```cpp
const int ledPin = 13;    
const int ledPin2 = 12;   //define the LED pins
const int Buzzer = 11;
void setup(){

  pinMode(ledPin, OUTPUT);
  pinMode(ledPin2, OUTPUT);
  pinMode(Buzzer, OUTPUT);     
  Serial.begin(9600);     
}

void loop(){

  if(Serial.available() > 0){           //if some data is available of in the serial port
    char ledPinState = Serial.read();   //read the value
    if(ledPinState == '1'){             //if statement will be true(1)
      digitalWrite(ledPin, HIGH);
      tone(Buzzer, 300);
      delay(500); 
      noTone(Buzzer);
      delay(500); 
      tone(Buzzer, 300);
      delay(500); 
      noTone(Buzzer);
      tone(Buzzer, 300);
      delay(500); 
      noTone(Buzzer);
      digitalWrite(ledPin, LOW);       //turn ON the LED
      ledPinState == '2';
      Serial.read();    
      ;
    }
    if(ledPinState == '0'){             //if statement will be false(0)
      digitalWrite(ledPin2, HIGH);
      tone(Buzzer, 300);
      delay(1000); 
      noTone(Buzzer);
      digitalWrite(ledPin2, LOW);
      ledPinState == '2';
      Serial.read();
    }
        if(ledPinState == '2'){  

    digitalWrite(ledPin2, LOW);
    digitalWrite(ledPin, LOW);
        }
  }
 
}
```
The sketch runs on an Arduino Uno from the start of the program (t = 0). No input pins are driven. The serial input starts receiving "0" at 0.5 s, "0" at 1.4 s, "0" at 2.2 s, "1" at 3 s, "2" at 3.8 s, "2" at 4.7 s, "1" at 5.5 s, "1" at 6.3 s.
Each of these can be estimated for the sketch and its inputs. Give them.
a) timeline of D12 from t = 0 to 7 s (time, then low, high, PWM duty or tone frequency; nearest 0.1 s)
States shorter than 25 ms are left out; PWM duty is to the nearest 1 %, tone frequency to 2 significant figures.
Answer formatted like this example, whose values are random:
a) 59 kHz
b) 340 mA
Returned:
a) 0 s low; 0.5 s high; 1.5 s low; 2.2 s high; 3.2 s low
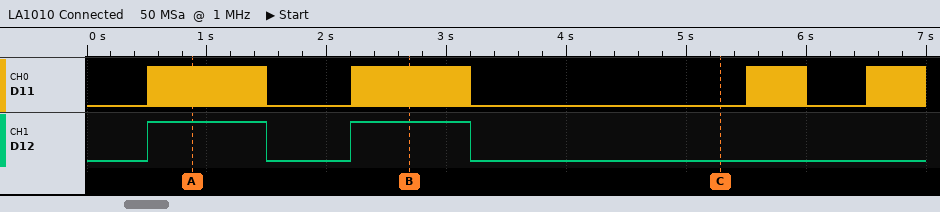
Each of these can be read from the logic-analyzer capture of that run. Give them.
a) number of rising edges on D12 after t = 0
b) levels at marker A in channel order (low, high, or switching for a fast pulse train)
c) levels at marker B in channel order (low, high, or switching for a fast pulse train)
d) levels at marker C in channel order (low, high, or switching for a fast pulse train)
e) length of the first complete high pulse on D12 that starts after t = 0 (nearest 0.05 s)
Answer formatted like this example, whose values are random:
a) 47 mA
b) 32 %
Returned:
a) 2
b) D11 switching, D12 high
c) D11 switching, D12 high
d) D11 low, D12 low
e) 1.00 s
